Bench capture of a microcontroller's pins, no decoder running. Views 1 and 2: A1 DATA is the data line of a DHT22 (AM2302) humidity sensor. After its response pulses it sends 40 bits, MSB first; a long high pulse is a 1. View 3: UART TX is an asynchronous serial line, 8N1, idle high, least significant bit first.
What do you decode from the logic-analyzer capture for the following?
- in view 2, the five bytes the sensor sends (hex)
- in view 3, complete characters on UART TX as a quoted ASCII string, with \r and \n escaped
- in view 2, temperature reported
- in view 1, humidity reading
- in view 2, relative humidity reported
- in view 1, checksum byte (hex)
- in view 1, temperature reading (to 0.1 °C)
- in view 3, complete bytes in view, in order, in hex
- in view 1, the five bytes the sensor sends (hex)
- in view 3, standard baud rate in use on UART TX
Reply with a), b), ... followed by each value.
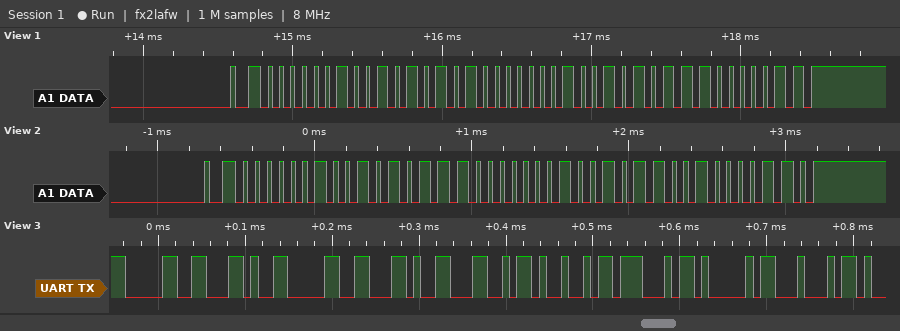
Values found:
a) 02 57 01 2C 86
b) "0,0,LIGAD"
c) 30.0 °C
d) 59.7 %
e) 59.9 %
f) 0x83
g) 29.9 °C
h) 30 2C 30 2C 4C 49 47 41 44
i) 02 55 01 2B 83
j) 115200 baud
